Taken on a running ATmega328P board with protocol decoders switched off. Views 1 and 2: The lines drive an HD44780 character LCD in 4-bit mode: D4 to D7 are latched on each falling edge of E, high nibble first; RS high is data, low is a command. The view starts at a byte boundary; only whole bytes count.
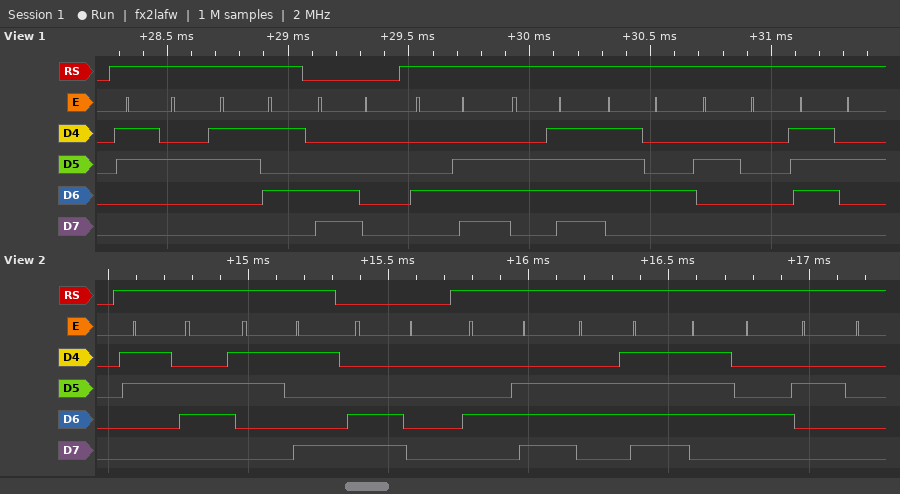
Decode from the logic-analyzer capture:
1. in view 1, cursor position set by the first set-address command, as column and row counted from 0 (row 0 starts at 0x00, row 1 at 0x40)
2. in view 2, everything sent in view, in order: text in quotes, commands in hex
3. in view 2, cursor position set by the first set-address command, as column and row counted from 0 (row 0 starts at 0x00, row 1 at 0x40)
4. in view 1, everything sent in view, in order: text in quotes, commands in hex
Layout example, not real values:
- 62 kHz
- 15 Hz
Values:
- column 0, row 1
- "69" 0xC0 "Not "
- column 0, row 1
- "25" 0xC0 "Not r"
